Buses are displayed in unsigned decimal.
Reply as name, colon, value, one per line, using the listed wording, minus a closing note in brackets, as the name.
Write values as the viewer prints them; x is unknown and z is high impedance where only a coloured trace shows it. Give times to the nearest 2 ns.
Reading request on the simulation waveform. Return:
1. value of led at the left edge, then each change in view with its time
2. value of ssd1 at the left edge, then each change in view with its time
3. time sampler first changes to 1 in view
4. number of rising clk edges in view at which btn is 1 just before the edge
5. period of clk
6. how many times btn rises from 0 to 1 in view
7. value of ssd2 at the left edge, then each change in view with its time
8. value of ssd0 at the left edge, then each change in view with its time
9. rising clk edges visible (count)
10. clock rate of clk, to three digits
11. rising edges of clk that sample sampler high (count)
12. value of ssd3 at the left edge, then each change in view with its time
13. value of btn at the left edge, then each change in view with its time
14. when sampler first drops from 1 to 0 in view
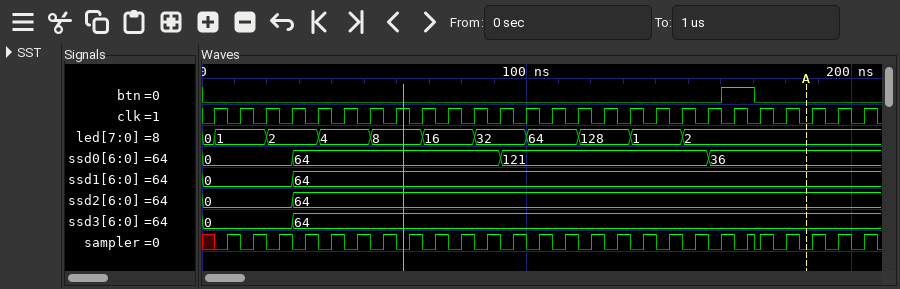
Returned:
value of led at the left edge, then each change in view with its time: 0, 1 at 4 ns, 2 at 20 ns, 4 at 36 ns, 8 at 52 ns, 16 at 68 ns, 32 at 84 ns, 64 at 100 ns, 128 at 116 ns, 1 at 132 ns, 2 at 148 ns
value of ssd1 at the left edge, then each change in view with its time: 0, 64 at 28 ns
time sampler first changes to 1 in view: 8 ns
number of rising clk edges in view at which btn is 1 just before the edge: 1
period of clk: 8 ns
how many times btn rises from 0 to 1 in view: 1
value of ssd2 at the left edge, then each change in view with its time: 0, 64 at 28 ns
value of ssd0 at the left edge, then each change in view with its time: 0, 64 at 28 ns, 121 at 92 ns, 36 at 156 ns
rising clk edges visible: 26
clock rate of clk, to three digits: 125 MHz
rising edges of clk that sample sampler high: 20
value of ssd3 at the left edge, then each change in view with its time: 0, 64 at 28 ns
value of btn at the left edge, then each change in view with its time: 0, 1 at 160 ns, 0 at 170 ns
when sampler first drops from 1 to 0 in view: 12 ns
